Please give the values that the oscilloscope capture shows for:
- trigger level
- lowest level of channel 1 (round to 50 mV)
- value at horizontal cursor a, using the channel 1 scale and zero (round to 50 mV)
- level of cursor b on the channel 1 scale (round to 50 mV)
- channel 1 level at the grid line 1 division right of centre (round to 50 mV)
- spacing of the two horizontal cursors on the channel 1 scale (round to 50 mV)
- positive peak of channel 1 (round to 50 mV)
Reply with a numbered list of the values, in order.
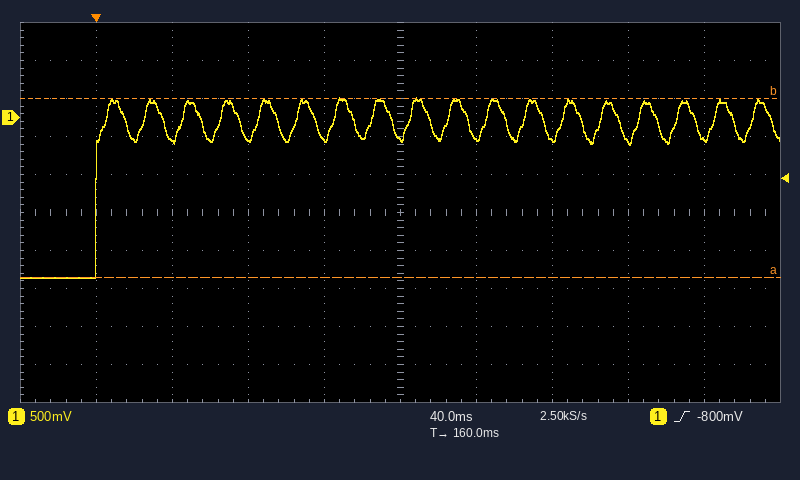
1. -800 mV
2. -2.10 V
3. -2.10 V
4. 250 mV
5. -250 mV
6. 2.35 V
7. 250 mV
